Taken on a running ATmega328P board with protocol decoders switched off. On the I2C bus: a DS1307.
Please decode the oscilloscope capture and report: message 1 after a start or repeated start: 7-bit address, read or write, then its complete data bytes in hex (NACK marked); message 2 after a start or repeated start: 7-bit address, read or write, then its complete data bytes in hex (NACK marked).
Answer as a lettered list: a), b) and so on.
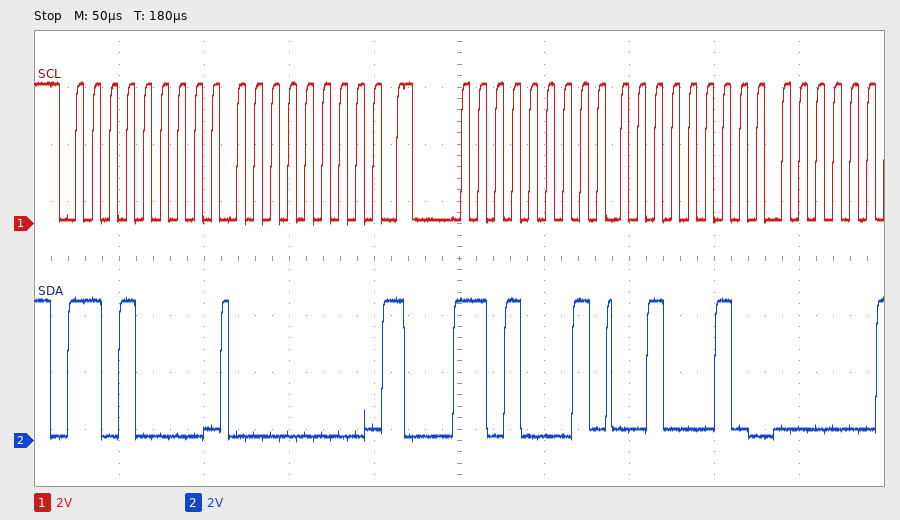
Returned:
a) 0x68 write: 00
b) 0x68 read: 22
